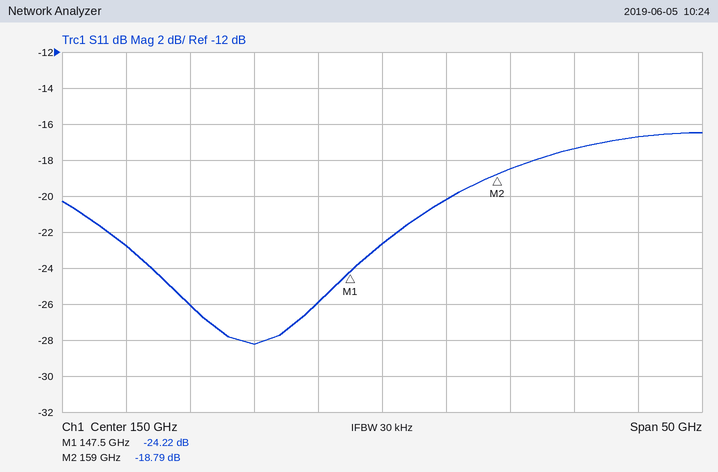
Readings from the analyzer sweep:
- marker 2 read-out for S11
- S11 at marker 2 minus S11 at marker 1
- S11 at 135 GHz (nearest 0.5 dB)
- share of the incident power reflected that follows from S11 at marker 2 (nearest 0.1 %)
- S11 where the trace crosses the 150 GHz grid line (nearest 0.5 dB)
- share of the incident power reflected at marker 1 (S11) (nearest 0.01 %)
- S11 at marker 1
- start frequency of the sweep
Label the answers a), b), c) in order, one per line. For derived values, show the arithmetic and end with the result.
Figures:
a) -18.79 dB
b) -18.79 − (-24.22) = 5.43 dB
c) -26.0 dB
d) 10^(-18.79/10) ≈ 1.3 %
e) -22.5 dB
f) 10^(-24.22/10) ≈ 0.38 %
g) -24.22 dB
h) 125 GHz
